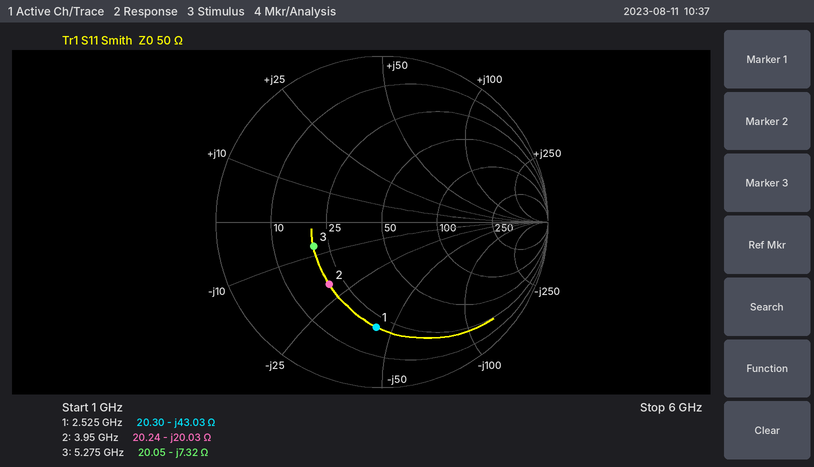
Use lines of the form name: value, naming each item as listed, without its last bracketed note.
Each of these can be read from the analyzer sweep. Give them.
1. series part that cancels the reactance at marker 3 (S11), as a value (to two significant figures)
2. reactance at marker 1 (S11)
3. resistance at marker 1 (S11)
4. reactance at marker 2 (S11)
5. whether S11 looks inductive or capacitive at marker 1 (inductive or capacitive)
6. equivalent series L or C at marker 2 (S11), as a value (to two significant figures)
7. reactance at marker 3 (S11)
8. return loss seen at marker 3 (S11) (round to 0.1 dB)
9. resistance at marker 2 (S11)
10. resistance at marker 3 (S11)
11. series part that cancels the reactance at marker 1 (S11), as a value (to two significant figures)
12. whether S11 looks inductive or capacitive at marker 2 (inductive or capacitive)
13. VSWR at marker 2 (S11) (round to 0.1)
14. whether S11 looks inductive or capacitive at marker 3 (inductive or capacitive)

series part that cancels the reactance at marker 3 (S11), as a value: 220 pH
reactance at marker 1: -43.03 Ω
resistance at marker 1: 20.30 Ω
reactance at marker 2: -20.03 Ω
whether S11 looks inductive or capacitive at marker 1: capacitive
equivalent series L or C at marker 2 (S11), as a value: 2.0 pF
reactance at marker 3: -7.32 Ω
return loss seen at marker 3 (S11): 7.2 dB
resistance at marker 2: 20.24 Ω
resistance at marker 3: 20.05 Ω
series part that cancels the reactance at marker 1 (S11), as a value: 2.7 nH
whether S11 looks inductive or capacitive at marker 2: capacitive
VSWR at marker 2 (S11): 2.9
whether S11 looks inductive or capacitive at marker 3: capacitive
